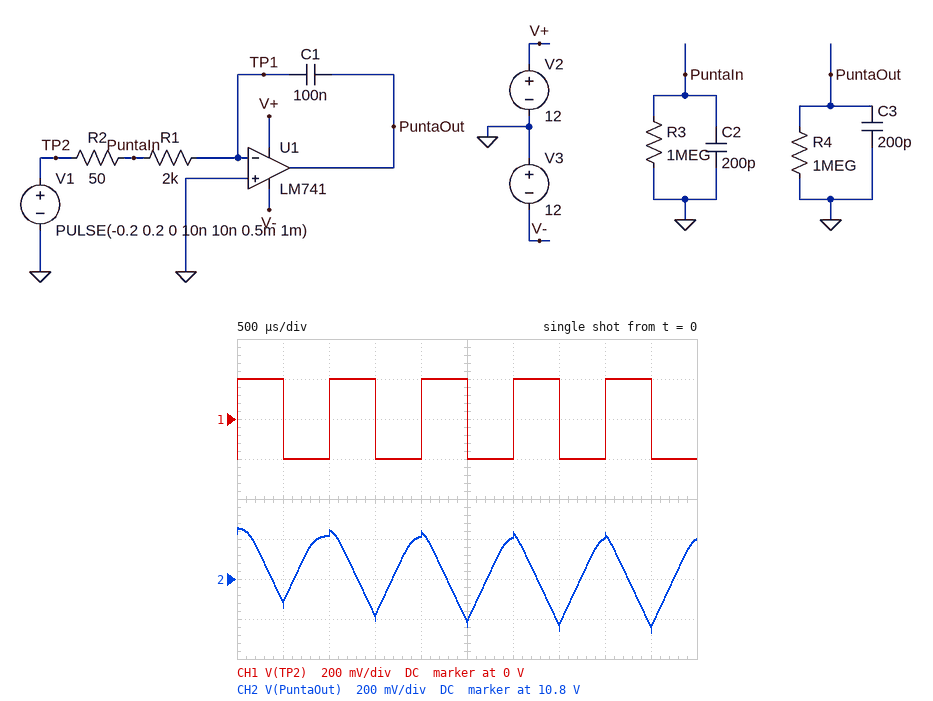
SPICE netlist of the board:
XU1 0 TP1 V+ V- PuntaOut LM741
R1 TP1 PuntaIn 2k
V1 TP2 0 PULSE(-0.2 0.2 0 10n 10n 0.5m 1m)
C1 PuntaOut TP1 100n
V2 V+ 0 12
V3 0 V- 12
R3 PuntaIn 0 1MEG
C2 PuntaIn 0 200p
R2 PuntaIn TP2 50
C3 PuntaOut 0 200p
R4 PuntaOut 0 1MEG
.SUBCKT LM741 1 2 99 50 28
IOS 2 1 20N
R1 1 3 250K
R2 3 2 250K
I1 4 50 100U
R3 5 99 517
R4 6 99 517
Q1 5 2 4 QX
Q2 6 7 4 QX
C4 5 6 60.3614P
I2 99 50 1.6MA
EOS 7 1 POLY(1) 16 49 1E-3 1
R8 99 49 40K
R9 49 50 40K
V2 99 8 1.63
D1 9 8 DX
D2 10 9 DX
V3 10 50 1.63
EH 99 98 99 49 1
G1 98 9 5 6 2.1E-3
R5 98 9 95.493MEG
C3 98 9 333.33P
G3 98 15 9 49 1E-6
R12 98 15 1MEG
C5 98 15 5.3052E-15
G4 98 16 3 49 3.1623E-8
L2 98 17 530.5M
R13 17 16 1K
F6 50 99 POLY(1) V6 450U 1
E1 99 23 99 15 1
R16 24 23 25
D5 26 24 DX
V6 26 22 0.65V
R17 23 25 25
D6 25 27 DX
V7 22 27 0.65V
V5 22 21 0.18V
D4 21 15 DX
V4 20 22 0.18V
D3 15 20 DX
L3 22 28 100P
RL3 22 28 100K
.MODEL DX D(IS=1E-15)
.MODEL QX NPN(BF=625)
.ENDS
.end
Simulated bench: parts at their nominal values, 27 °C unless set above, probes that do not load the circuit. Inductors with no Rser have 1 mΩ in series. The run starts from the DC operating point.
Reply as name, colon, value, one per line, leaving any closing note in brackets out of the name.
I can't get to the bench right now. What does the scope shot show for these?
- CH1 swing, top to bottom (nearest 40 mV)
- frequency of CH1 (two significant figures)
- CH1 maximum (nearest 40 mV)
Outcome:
CH1 swing, top to bottom: 400 mV
frequency of CH1: 1.0 kHz
CH1 maximum: 200 mV
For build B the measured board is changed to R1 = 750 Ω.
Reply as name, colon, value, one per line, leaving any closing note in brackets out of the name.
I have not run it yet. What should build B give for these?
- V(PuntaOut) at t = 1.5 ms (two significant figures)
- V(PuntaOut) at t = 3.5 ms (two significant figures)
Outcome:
V(PuntaOut) at t = 1.5 ms: 9.9 V
V(PuntaOut) at t = 3.5 ms: 9.8 V
